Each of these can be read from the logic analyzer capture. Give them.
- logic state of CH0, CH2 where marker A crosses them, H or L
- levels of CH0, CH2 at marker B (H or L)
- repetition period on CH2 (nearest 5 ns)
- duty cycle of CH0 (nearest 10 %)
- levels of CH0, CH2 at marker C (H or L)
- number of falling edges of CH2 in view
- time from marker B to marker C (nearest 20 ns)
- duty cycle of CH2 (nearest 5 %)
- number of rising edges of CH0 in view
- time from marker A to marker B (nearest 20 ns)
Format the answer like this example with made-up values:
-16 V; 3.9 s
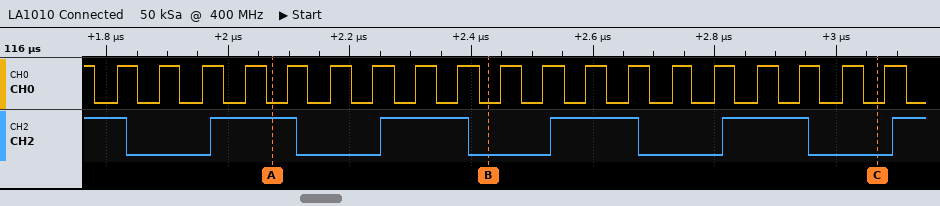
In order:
CH0=L, CH2=H; CH0=L, CH2=L; 280 ns; 50 %; CH0=L, CH2=L; 5; 640 ns; 50 %; 19; 360 ns
